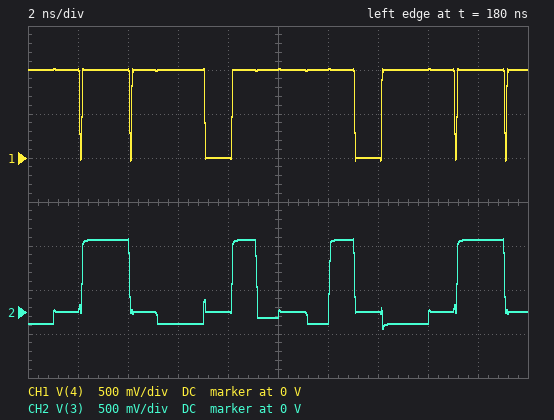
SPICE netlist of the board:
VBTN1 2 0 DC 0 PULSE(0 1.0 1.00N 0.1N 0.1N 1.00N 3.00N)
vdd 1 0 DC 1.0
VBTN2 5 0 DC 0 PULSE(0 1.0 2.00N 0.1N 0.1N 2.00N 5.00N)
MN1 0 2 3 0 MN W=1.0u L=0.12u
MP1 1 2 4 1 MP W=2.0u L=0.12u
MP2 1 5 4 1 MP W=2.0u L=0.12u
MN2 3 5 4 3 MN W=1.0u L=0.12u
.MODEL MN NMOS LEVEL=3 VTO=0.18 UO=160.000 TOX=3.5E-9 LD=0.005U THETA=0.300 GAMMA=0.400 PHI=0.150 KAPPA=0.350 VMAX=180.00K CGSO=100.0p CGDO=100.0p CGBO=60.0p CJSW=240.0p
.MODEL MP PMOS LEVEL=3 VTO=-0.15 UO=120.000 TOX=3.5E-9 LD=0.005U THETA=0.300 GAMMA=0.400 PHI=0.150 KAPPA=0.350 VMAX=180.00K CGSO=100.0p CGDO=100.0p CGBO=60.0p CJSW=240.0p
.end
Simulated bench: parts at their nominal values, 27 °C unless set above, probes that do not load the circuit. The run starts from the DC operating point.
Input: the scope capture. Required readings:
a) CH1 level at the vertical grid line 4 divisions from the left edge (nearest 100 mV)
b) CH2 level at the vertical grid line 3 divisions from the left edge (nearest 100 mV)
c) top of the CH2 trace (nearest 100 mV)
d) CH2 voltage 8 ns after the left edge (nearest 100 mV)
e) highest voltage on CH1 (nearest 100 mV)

0 V
-100 mV
800 mV
0 V
1.0 V
